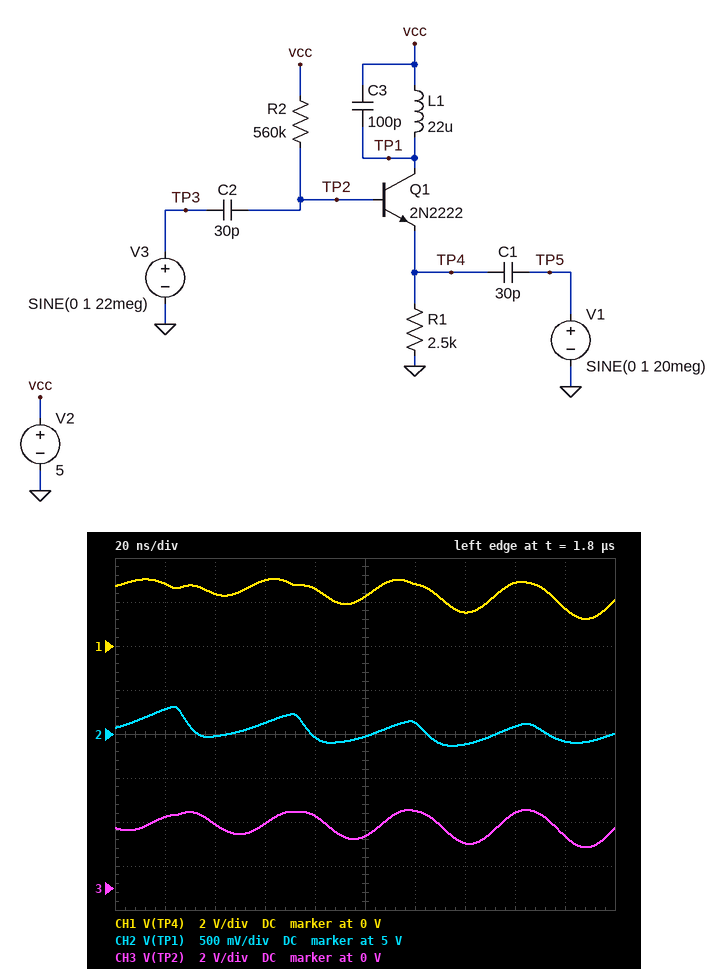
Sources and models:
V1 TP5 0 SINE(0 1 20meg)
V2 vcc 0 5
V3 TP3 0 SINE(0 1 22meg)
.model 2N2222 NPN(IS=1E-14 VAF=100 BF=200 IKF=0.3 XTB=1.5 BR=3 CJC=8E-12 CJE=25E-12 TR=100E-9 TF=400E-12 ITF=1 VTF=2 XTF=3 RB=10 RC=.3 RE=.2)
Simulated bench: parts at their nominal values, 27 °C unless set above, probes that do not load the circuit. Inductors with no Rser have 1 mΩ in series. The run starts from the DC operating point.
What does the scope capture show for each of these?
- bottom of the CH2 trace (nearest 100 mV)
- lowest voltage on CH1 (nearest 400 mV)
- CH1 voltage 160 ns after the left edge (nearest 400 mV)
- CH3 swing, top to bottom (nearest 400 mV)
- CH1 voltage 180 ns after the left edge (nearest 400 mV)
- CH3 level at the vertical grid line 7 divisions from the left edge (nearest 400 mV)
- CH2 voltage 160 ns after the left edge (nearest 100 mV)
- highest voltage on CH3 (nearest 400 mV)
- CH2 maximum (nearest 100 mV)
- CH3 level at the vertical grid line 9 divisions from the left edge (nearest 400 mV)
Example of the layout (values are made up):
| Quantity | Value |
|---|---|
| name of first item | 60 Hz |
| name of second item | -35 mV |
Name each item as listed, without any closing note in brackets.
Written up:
| Quantity | Value |
|---|---|
| bottom of the CH2 trace | 4.9 V |
| lowest voltage on CH1 | 1.2 V |
| CH1 voltage 160 ns after the left edge | 2.8 V |
| CH3 swing, top to bottom | 1.6 V |
| CH1 voltage 180 ns after the left edge | 1.6 V |
| CH3 level at the vertical grid line 7 divisions from the left edge | 2.0 V |
| CH2 voltage 160 ns after the left edge | 5.1 V |
| highest voltage on CH3 | 3.6 V |
| CH2 maximum | 5.3 V |
| CH3 level at the vertical grid line 9 divisions from the left edge | 2.4 V |
